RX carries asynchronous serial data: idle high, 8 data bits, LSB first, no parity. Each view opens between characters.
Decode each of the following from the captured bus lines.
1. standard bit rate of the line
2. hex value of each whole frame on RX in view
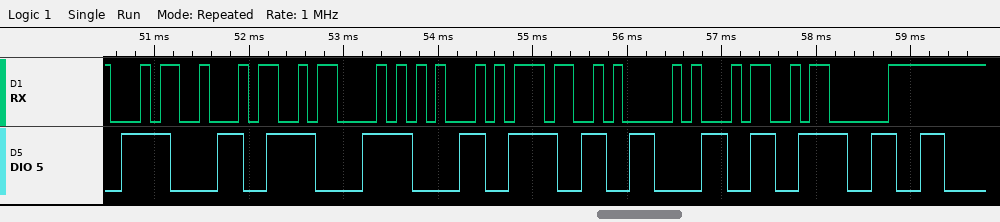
9600 baud
34, 34, 43, 45, 37, 41, 34, 03
